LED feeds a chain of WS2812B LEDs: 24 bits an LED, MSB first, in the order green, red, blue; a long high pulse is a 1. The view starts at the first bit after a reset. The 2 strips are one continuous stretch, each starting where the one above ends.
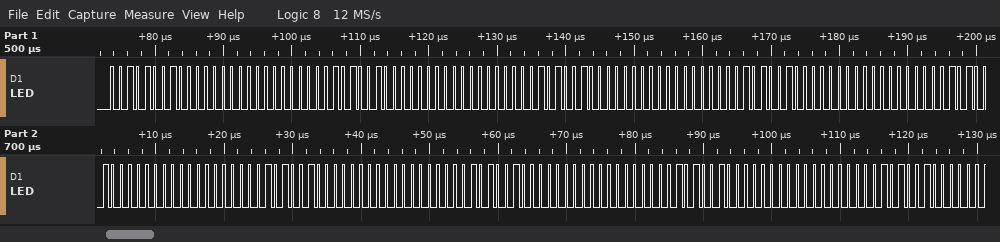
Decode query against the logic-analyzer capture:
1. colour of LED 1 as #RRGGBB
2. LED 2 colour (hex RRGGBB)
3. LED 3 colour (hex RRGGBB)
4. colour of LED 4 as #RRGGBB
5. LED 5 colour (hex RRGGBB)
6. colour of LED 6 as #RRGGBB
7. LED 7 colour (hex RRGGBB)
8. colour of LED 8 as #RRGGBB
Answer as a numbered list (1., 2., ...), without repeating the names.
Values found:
1. #002900
2. #002900
3. #002900
4. #002900
5. #002900
6. #002900
7. #002900
8. #002900
